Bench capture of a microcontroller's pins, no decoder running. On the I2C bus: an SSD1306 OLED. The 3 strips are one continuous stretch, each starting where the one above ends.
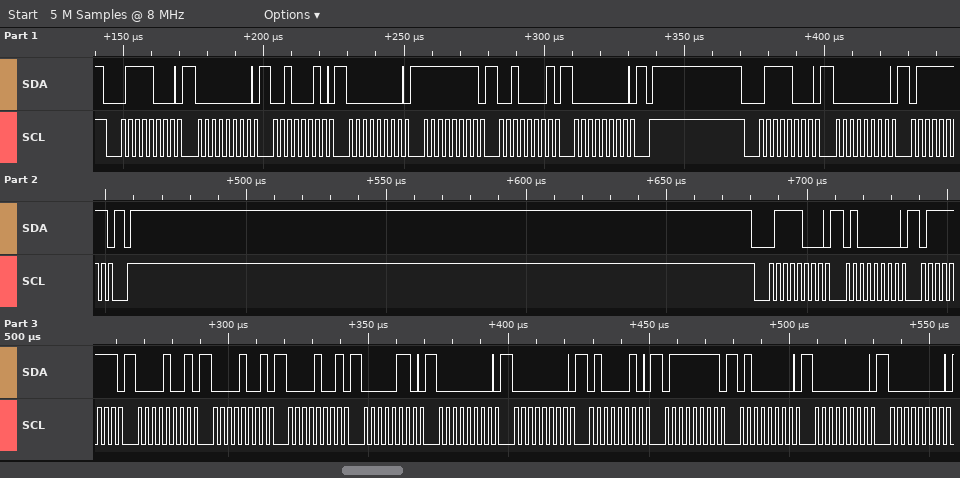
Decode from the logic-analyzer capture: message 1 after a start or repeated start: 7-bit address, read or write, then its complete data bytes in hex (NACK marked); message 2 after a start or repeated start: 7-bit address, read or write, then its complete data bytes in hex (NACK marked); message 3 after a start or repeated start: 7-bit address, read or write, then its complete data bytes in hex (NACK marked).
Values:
0x3C write: 00 22 00 FF 21 00
0x3C write: 00 7F
0x3C write: 40 7F 09 09 09 06 00 00 42 7F 40 00 00
